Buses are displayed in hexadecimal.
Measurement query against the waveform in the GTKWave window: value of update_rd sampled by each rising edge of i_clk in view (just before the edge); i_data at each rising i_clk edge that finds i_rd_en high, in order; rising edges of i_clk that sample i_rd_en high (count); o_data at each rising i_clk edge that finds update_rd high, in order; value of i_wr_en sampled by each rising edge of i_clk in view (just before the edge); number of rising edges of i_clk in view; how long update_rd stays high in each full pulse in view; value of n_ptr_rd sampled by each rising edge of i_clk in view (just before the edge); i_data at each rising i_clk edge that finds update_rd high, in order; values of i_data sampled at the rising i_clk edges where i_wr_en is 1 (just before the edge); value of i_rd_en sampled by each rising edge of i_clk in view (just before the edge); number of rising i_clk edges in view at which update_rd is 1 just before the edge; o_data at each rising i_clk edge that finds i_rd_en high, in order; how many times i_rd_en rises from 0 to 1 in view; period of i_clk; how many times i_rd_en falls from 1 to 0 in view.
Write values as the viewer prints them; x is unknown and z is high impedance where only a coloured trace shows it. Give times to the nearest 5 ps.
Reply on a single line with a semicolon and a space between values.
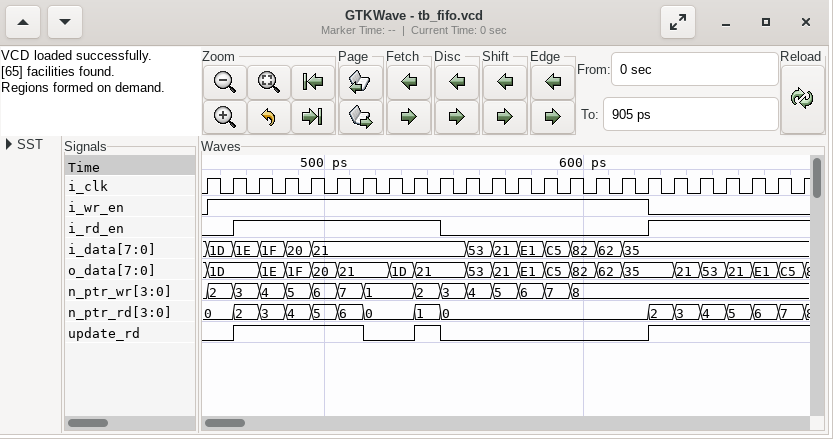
0 0 1 1 1 1 1 0 0 1 0 0 0 0 0 0 0 0 1 1 1 1 1 1; 1E, 1F, 20, 21, 21, 21, 21, 21, 35, 35, 35, 35, 35, 35; 14; 1D, 1E, 1F, 20, 21, 21, 35, 21, 53, 21, E1, C5; 0 1 1 1 1 1 1 1 1 1 1 1 1 1 1 1 1 1 0 0 0 0 0 0; 24; 50 ps, 10 ps; 0, 0, 2, 3, 4, 5, 6, 0, 0, 1, 0, 0, 0, 0, 0, 0, 0, 0, 2, 3, 4, 5, 6, 7; 1E, 1F, 20, 21, 21, 21, 35, 35, 35, 35, 35, 35; 1D, 1E, 1F, 20, 21, 21, 21, 21, 21, 21, 53, 21, E1, C5, 82, 62, 35; 0 0 1 1 1 1 1 1 1 1 0 0 0 0 0 0 0 0 1 1 1 1 1 1; 12; 1D, 1E, 1F, 20, 21, 21, 1D, 21, 35, 21, 53, 21, E1, C5; 2; 10 ps; 1
